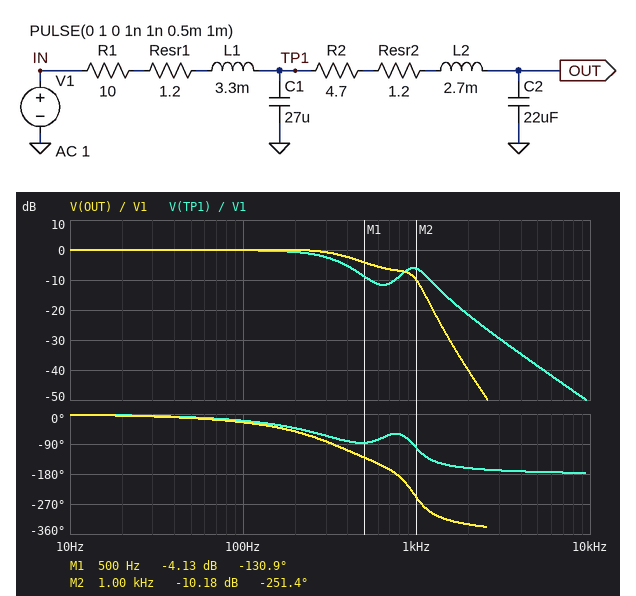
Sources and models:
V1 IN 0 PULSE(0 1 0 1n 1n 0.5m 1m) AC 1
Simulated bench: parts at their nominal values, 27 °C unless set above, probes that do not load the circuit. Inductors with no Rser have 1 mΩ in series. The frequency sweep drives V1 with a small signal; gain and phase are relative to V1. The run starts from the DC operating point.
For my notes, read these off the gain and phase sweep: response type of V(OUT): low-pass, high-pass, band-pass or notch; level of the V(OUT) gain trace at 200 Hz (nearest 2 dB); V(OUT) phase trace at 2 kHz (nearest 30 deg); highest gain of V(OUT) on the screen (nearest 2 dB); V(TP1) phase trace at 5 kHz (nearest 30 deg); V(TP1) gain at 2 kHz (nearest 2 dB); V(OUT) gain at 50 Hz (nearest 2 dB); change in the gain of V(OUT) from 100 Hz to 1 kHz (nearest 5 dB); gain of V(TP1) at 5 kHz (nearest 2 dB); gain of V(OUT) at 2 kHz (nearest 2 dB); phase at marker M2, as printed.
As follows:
low-pass
0 dB
-330 deg
0 dB
-180 deg
-22 dB
0 dB
-10 dB
-38 dB
-40 dB
-251.4 deg
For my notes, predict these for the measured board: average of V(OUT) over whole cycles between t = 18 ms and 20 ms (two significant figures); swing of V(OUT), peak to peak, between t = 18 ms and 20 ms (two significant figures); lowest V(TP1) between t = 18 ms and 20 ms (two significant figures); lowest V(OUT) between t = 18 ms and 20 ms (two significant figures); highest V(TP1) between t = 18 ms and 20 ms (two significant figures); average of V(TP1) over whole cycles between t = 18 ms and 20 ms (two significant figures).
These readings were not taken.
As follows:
500 mV
390 mV
180 mV
300 mV
820 mV
500 mV
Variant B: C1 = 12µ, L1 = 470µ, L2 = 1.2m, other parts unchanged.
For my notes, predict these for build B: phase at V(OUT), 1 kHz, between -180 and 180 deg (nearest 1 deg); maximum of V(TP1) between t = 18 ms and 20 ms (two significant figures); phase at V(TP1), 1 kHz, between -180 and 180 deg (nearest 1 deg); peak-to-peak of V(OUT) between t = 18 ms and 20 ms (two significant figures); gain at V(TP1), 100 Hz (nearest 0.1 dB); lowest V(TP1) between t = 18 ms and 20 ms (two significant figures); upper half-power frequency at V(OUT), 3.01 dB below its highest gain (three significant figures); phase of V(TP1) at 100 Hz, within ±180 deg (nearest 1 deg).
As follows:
-118 deg
730 mV
-25 deg
530 mV
-0.3 dB
270 mV
429 Hz
-13 deg
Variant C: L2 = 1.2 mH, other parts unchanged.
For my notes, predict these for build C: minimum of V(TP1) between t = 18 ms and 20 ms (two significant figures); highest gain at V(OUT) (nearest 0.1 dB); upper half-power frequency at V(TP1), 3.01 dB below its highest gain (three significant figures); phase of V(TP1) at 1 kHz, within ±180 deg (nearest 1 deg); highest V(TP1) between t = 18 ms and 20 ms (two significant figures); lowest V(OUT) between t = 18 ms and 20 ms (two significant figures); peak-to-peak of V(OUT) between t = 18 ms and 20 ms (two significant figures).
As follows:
370 mV
0 dB
354 Hz
-95 deg
630 mV
350 mV
290 mV
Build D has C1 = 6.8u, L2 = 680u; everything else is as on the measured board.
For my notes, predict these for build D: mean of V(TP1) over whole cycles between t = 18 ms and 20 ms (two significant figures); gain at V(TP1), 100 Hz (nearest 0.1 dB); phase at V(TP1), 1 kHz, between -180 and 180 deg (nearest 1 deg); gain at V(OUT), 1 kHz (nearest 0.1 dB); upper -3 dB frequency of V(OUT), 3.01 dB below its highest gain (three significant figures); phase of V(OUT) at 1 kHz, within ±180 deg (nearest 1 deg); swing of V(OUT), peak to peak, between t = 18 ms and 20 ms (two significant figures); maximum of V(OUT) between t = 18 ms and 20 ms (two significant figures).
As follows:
500 mV
0 dB
-87 deg
-11.4 dB
533 Hz
-150 deg
370 mV
680 mV
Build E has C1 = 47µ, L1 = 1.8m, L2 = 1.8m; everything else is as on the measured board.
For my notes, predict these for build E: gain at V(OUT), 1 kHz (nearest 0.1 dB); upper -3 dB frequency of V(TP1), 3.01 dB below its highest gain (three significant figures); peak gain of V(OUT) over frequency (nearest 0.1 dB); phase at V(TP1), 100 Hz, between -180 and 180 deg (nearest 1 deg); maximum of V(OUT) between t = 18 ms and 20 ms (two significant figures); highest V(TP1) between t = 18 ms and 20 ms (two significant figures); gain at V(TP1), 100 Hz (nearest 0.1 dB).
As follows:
-11.3 dB
231 Hz
0 dB
-27 deg
670 mV
680 mV
-0.7 dB
